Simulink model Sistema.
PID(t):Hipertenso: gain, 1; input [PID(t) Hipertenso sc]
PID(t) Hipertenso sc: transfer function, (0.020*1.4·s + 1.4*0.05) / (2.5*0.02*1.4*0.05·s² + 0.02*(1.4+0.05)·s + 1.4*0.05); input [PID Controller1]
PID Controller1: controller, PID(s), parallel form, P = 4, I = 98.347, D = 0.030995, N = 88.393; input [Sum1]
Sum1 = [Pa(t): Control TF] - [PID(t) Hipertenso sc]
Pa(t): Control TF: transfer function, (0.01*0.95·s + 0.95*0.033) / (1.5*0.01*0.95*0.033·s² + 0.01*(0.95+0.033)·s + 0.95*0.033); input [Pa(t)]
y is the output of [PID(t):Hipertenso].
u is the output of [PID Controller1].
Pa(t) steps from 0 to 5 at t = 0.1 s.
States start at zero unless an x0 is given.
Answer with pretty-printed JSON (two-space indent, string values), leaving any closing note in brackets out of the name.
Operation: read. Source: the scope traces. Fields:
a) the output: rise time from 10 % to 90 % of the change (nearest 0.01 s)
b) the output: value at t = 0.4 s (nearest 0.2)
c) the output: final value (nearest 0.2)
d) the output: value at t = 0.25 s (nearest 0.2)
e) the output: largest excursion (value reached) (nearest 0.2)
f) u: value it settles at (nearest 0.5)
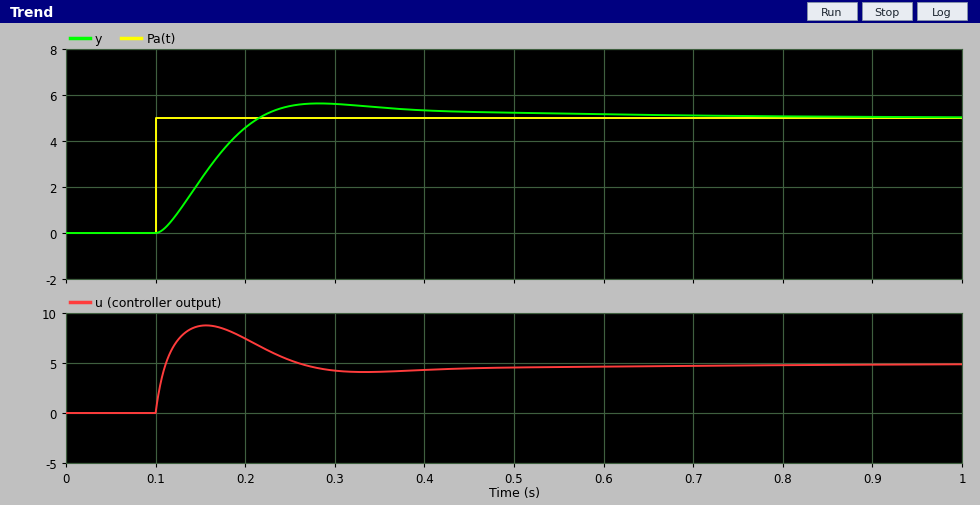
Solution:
{
  "the output: rise time from 10 % to 90 % of the change": "0.08 s",
  "the output: value at t = 0.4 s": "5.4",
  "the output: final value": "5.0",
  "the output: value at t = 0.25 s": "5.6",
  "the output: largest excursion (value reached)": "5.6",
  "u: value it settles at": "5.0"
}
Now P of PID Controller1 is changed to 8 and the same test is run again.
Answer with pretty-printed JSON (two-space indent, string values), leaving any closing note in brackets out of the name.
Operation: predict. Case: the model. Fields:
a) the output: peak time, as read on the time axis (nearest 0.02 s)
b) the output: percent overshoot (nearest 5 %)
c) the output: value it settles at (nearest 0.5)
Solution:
{
  "the output: peak time, as read on the time axis": "0.32 s",
  "the output: percent overshoot": "10 %",
  "the output: value it settles at": "5.0"
}
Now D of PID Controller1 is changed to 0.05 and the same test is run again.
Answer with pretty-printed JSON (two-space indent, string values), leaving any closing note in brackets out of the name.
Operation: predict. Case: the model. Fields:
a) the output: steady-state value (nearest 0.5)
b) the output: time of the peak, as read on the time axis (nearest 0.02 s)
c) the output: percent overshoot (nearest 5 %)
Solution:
{
  "the output: steady-state value": "5.0",
  "the output: time of the peak, as read on the time axis": "0.28 s",
  "the output: percent overshoot": "15 %"
}
